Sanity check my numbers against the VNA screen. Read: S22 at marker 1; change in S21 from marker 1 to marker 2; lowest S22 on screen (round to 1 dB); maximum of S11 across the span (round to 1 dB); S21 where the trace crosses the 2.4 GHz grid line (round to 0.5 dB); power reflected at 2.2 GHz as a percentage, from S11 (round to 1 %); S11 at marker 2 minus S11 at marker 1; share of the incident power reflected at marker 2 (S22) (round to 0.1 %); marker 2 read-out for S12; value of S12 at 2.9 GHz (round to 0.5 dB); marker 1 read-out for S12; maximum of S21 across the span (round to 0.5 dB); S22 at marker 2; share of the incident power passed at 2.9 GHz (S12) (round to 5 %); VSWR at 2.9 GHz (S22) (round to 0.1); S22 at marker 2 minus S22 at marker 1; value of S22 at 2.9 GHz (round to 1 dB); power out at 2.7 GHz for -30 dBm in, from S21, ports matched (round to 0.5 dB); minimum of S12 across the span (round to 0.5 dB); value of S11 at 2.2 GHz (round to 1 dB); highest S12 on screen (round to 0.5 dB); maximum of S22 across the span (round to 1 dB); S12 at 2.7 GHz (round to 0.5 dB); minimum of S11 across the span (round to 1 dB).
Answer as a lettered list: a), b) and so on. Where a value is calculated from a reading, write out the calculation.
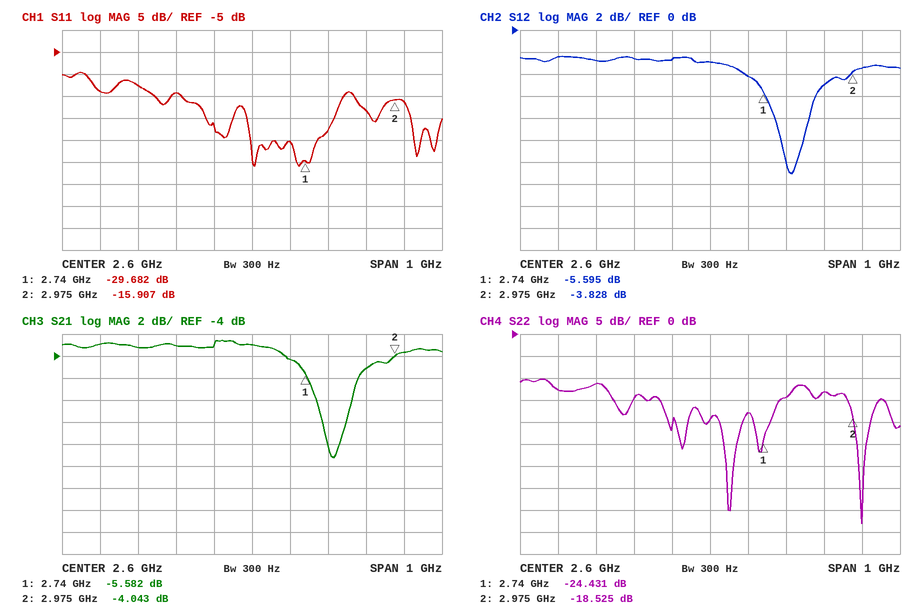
a) -24.431 dB
b) -4.043 − (-5.582) = 1.539 dB
c) -43 dB
d) -10 dB
e) -3.0 dB
f) 10^(-14/10) ≈ 4 %
g) -15.907 − (-29.682) = 13.775 dB
h) 10^(-18.525/10) ≈ 1.4 %
i) -3.828 dB
j) -5.0 dB
k) -5.595 dB
l) -2.5 dB
m) -18.525 dB
n) 10^(-5/10) ≈ 31.6 %, so 30 % to the nearest 5 %
o) |Γ| = 10^(-13/20) = 0.2239; VSWR = (1 + 0.2239)/(1 − 0.2239) ≈ 1.6
p) -18.525 − (-24.431) = 5.906 dB
q) -13 dB
r) -30 dBm + (-4.5 dB) = -34.5 dBm
s) -13.0 dB
t) -14 dB
u) -2.5 dB
v) -10 dB
w) -4.0 dB
x) -31 dB
